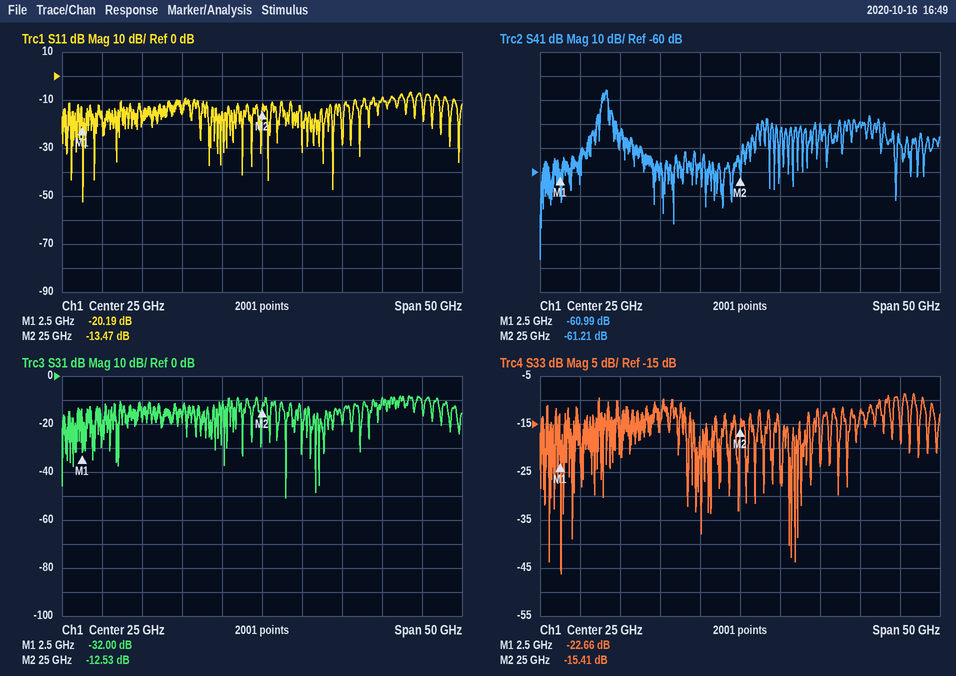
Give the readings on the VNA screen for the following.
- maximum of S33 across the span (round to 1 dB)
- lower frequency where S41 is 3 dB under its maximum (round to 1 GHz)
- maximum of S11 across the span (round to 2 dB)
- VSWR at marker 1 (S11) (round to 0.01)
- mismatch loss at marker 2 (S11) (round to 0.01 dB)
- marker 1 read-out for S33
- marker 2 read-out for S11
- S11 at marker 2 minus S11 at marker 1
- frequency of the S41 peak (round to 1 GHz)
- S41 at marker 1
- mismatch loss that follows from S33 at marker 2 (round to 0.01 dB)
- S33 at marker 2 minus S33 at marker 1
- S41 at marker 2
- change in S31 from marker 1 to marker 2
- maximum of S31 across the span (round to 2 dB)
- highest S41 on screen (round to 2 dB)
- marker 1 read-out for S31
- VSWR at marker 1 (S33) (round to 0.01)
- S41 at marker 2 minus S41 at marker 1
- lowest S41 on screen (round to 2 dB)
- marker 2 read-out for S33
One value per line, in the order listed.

-9 dB
8 GHz
-6 dB
1.22
0.20 dB
-22.66 dB
-13.47 dB
6.72 dB
8 GHz
-60.99 dB
0.13 dB
7.25 dB
-61.21 dB
19.47 dB
-8 dB
-26 dB
-32.00 dB
1.16
-0.22 dB
-96 dB
-15.41 dB
